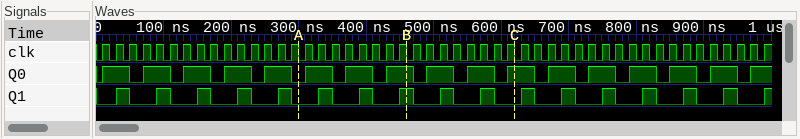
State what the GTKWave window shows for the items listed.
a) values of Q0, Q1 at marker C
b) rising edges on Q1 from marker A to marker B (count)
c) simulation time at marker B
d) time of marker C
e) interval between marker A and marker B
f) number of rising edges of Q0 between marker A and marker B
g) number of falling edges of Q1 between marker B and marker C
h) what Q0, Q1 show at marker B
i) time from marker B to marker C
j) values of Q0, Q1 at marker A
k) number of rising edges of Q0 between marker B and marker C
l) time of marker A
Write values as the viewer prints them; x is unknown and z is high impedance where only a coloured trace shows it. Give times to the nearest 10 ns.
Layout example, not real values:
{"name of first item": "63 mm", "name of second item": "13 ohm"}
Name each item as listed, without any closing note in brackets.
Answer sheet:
{"values of Q0, Q1 at marker C": "Q0=1, Q1=0", "rising edges on Q1 from marker A to marker B": "3", "simulation time at marker B": "460 ns", "time of marker C": "620 ns", "interval between marker A and marker B": "160 ns", "number of rising edges of Q0 between marker A and marker B": "3", "number of falling edges of Q1 between marker B and marker C": "3", "what Q0, Q1 show at marker B": "Q0=1, Q1=1", "time from marker B to marker C": "160 ns", "values of Q0, Q1 at marker A": "Q0=0, Q1=0", "number of rising edges of Q0 between marker B and marker C": "3", "time of marker A": "300 ns"}
